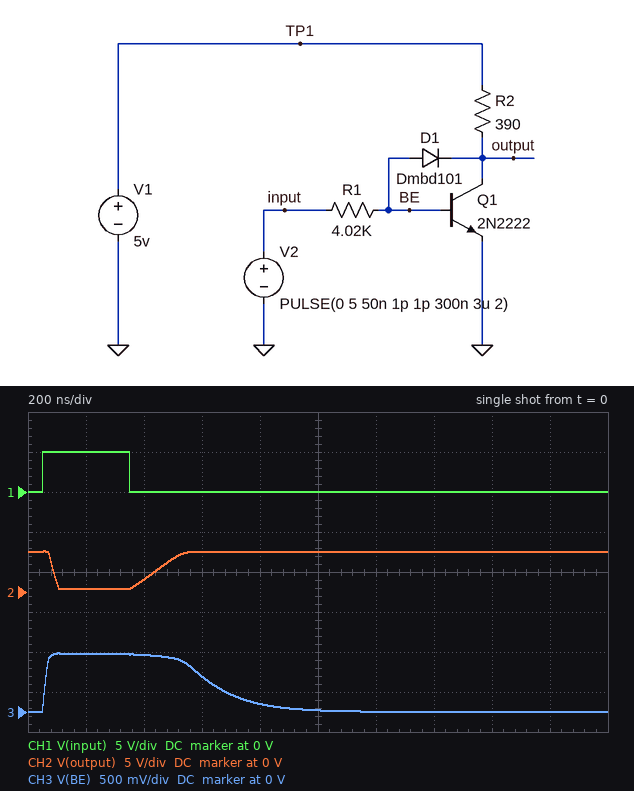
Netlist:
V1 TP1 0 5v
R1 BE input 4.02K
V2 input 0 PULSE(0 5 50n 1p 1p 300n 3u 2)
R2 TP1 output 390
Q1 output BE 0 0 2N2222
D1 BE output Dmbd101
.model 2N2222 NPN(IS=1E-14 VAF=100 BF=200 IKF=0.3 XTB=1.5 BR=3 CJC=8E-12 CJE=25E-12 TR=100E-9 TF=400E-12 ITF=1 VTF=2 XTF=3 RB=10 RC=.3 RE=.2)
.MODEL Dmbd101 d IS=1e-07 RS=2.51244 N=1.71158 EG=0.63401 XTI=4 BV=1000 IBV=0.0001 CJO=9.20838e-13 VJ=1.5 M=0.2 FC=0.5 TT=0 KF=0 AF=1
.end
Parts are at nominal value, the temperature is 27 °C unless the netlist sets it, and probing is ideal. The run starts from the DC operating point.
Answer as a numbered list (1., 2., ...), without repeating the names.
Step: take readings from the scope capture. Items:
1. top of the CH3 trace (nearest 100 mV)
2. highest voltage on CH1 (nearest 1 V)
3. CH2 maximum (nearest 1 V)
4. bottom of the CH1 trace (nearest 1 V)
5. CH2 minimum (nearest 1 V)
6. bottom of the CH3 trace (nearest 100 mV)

1. 700 mV
2. 5 V
3. 5 V
4. 0 V
5. 0 V
6. 0 V
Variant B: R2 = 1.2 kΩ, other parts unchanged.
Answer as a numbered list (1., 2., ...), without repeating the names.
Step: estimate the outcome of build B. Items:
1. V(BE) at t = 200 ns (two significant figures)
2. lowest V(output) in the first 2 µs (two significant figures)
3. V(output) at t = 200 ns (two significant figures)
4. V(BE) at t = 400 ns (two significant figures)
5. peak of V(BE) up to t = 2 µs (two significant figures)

1. 700 mV
2. 280 mV
3. 290 mV
4. 680 mV
5. 710 mV
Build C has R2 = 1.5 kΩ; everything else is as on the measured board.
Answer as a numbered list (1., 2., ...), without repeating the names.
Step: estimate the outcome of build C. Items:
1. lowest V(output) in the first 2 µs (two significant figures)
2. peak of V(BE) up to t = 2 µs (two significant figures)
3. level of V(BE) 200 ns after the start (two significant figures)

1. 280 mV
2. 700 mV
3. 690 mV
